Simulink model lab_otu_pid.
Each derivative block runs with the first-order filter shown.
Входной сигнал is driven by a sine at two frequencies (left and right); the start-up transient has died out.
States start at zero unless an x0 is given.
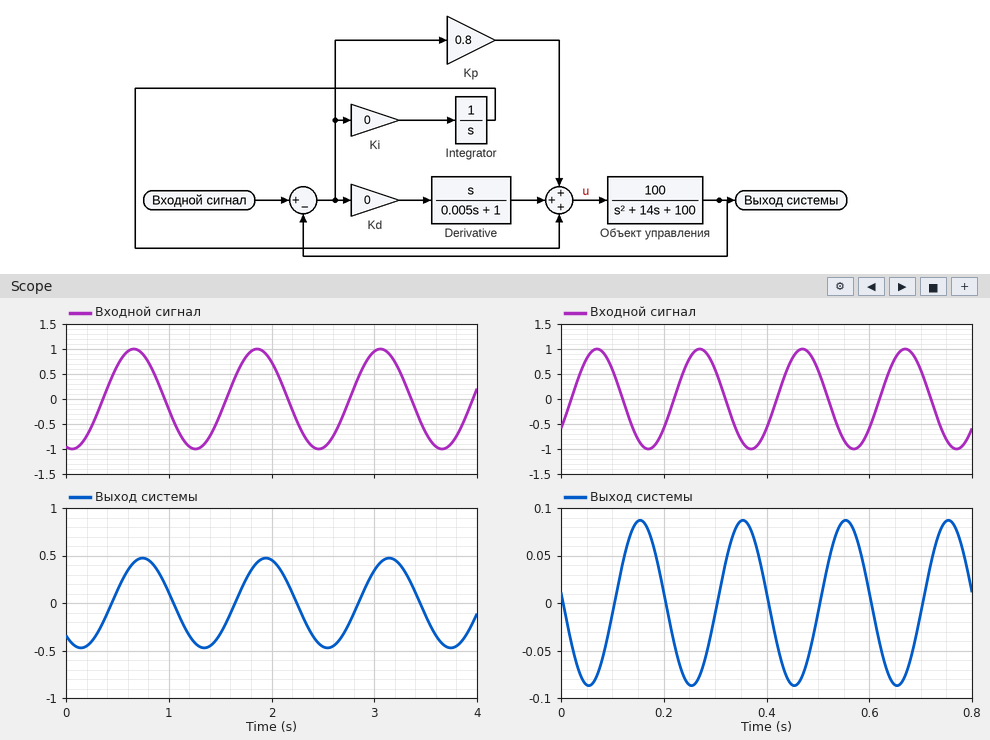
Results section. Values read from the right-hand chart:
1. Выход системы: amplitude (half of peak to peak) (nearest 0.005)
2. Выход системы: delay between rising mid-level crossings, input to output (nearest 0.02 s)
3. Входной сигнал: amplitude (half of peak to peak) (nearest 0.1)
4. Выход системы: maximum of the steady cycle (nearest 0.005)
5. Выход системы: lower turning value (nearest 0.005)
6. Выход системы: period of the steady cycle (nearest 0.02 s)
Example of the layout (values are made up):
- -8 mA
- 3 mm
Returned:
- 0.085
- 0.08 s
- 1.0
- 0.085
- -0.085
- 0.20 s
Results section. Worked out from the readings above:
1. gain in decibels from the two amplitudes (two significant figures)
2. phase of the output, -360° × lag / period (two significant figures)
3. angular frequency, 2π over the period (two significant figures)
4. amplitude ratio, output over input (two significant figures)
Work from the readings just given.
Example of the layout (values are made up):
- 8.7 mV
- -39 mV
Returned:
- -21 dB
- -140°
- 31 rad/s
- 0.085
